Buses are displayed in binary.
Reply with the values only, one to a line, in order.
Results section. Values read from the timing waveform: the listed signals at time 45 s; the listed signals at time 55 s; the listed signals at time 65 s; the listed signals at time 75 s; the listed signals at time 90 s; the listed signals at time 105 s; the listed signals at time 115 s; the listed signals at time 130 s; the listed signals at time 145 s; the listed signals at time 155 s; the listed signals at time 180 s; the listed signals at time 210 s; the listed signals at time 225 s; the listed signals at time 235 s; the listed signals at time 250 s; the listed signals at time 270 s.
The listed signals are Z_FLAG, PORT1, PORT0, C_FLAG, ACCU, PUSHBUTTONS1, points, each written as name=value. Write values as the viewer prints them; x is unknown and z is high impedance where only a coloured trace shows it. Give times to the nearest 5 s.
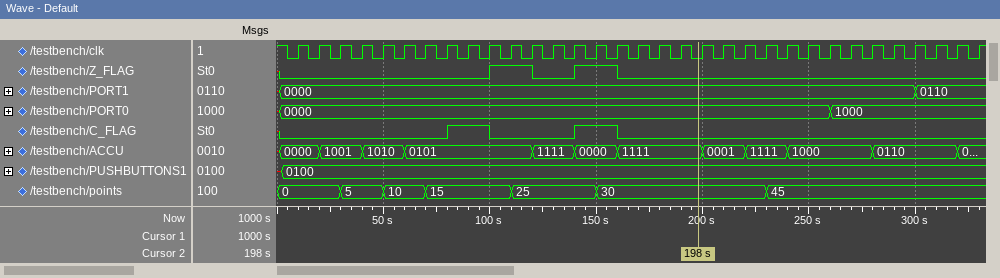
Z_FLAG=0, PORT1=0000, PORT0=0000, C_FLAG=0, ACCU=1010, PUSHBUTTONS1=0100, points=5
Z_FLAG=0, PORT1=0000, PORT0=0000, C_FLAG=0, ACCU=1010, PUSHBUTTONS1=0100, points=10
Z_FLAG=0, PORT1=0000, PORT0=0000, C_FLAG=0, ACCU=0101, PUSHBUTTONS1=0100, points=10
Z_FLAG=0, PORT1=0000, PORT0=0000, C_FLAG=0, ACCU=0101, PUSHBUTTONS1=0100, points=15
Z_FLAG=0, PORT1=0000, PORT0=0000, C_FLAG=1, ACCU=0101, PUSHBUTTONS1=0100, points=15
Z_FLAG=1, PORT1=0000, PORT0=0000, C_FLAG=0, ACCU=0101, PUSHBUTTONS1=0100, points=15
Z_FLAG=1, PORT1=0000, PORT0=0000, C_FLAG=0, ACCU=0101, PUSHBUTTONS1=0100, points=25
Z_FLAG=0, PORT1=0000, PORT0=0000, C_FLAG=0, ACCU=1111, PUSHBUTTONS1=0100, points=25
Z_FLAG=1, PORT1=0000, PORT0=0000, C_FLAG=1, ACCU=0000, PUSHBUTTONS1=0100, points=25
Z_FLAG=1, PORT1=0000, PORT0=0000, C_FLAG=1, ACCU=0000, PUSHBUTTONS1=0100, points=30
Z_FLAG=0, PORT1=0000, PORT0=0000, C_FLAG=0, ACCU=1111, PUSHBUTTONS1=0100, points=30
Z_FLAG=0, PORT1=0000, PORT0=0000, C_FLAG=0, ACCU=0001, PUSHBUTTONS1=0100, points=30
Z_FLAG=0, PORT1=0000, PORT0=0000, C_FLAG=0, ACCU=1111, PUSHBUTTONS1=0100, points=30
Z_FLAG=0, PORT1=0000, PORT0=0000, C_FLAG=0, ACCU=1111, PUSHBUTTONS1=0100, points=45
Z_FLAG=0, PORT1=0000, PORT0=0000, C_FLAG=0, ACCU=1000, PUSHBUTTONS1=0100, points=45
Z_FLAG=0, PORT1=0000, PORT0=1000, C_FLAG=0, ACCU=1000, PUSHBUTTONS1=0100, points=45
